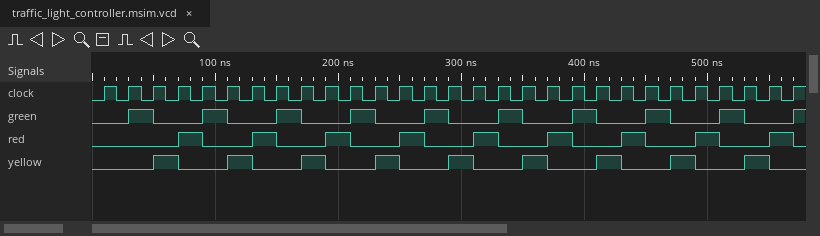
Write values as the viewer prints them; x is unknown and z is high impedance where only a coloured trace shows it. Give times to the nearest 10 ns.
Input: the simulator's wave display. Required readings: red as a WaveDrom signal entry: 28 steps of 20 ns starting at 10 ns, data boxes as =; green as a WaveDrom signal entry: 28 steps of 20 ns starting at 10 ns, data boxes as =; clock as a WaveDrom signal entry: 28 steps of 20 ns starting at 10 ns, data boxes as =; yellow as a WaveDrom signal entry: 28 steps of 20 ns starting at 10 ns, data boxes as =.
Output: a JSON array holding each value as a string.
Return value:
["{name: 'red', wave: '0..10.10.10.10.10.10.10.10.1'}", "{name: 'green', wave: '010.10.10.10.10.10.10.10.10.'}", "{name: 'clock', wave: 'p...........................'}", "{name: 'yellow', wave: '0.10.10.10.10.10.10.10.10.10'}"]
